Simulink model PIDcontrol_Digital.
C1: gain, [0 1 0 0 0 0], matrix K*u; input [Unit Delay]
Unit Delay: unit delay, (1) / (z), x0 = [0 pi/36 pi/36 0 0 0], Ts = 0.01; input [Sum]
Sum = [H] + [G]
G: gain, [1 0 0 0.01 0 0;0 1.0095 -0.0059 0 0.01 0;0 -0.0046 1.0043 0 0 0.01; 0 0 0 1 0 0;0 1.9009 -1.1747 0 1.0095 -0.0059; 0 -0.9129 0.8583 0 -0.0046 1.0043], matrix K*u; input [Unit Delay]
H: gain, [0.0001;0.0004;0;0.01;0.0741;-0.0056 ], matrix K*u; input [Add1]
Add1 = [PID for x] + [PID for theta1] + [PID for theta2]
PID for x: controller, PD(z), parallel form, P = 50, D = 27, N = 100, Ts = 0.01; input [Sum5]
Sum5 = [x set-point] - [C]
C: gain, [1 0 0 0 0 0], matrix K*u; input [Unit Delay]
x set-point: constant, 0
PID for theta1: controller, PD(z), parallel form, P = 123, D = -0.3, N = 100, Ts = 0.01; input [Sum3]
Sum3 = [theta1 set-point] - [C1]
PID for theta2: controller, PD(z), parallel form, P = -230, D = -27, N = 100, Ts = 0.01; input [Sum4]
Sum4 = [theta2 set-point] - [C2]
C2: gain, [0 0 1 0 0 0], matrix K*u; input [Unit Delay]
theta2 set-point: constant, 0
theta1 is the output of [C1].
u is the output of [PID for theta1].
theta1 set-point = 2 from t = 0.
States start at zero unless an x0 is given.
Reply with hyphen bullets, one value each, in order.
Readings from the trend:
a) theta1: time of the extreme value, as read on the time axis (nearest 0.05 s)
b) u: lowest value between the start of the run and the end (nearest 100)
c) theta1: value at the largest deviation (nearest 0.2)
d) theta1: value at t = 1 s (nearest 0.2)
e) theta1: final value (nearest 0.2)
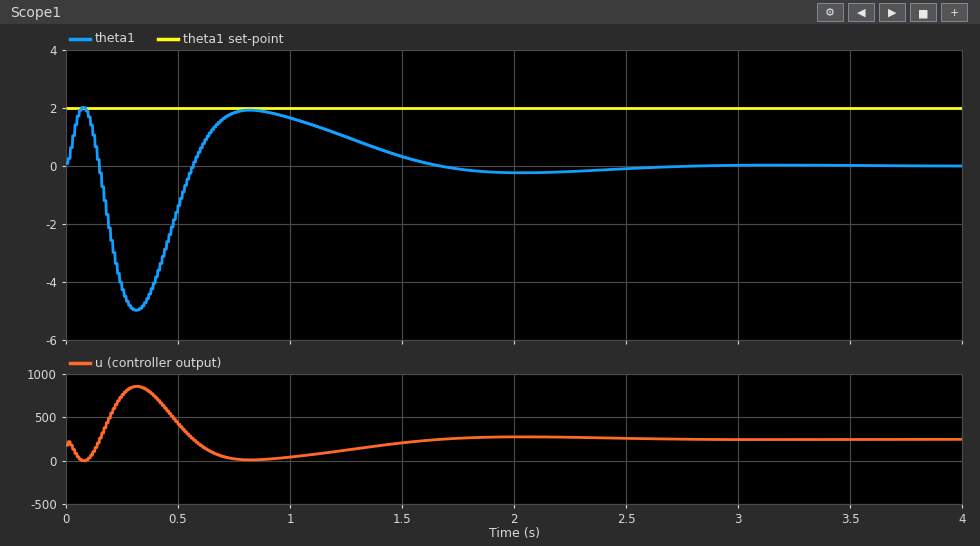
- 0.30 s
- 0
- -5.0
- 1.6
- 0.0
